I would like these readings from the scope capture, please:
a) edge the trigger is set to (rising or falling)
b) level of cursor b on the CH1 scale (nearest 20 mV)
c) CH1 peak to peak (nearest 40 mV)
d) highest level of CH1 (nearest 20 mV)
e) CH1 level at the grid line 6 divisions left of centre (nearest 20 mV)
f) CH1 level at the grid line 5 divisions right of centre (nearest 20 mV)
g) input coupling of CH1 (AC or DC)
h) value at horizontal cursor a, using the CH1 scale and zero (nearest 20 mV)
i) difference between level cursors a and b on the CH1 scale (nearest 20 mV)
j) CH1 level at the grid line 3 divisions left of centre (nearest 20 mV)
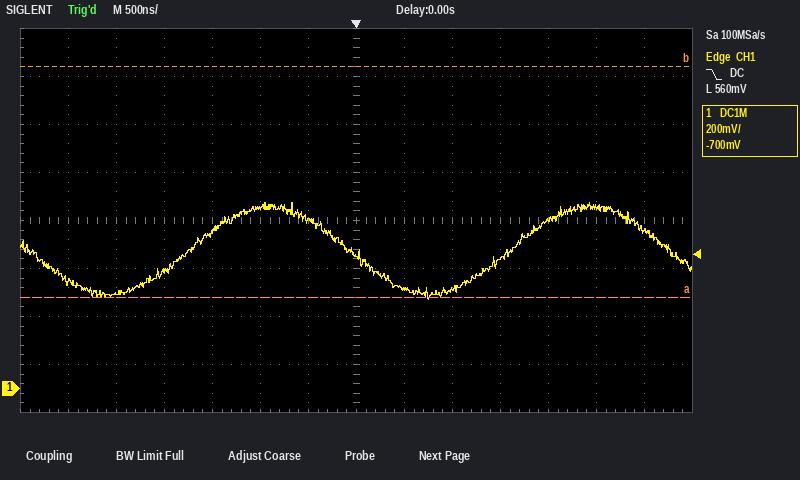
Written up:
falling
1.34 V
400 mV
780 mV
440 mV
760 mV
DC
380 mV
960 mV
640 mV
